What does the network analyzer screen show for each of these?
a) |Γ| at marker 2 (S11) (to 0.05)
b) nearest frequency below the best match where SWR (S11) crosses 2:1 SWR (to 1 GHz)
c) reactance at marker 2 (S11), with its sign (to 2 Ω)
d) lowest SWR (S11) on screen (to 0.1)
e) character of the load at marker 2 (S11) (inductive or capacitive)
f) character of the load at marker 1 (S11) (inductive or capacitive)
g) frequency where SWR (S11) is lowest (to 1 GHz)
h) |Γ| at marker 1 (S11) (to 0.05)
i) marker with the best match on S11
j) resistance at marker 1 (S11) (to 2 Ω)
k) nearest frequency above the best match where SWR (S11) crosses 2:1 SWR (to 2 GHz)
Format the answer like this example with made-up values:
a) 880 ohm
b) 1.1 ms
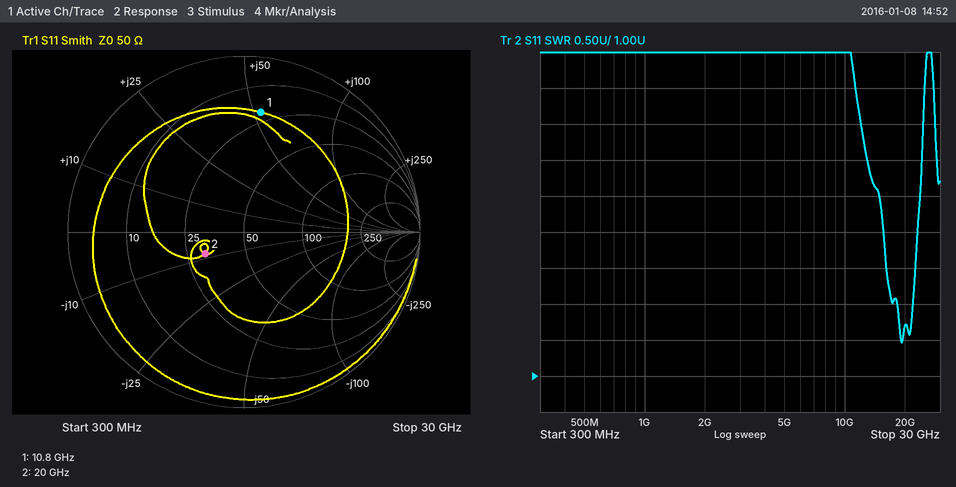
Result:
a) 0.25
b) 18 GHz
c) -8 Ω
d) 1.5
e) capacitive
f) inductive
g) 19 GHz
h) 0.70
i) marker 2
j) 20 Ω
k) 22 GHz
